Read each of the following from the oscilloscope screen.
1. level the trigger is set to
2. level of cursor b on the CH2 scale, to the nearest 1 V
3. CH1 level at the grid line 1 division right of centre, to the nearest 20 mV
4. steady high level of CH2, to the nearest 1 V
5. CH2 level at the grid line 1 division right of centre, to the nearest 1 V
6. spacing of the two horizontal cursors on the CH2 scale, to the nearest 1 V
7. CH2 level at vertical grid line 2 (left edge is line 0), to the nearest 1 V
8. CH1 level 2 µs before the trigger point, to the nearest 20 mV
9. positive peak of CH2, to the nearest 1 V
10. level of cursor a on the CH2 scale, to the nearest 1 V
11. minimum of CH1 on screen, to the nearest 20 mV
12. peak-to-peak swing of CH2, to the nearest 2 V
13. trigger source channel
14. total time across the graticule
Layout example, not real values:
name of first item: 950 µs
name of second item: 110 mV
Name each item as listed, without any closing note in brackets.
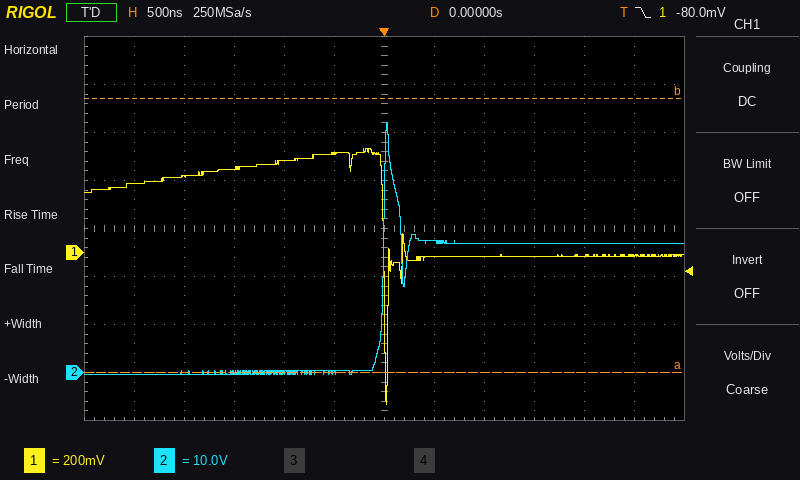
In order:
level the trigger is set to: -80.0 mV
level of cursor b on the CH2 scale, to the nearest 1 V: 57 V
CH1 level at the grid line 1 division right of centre, to the nearest 20 mV: -20 mV
steady high level of CH2, to the nearest 1 V: 27 V
CH2 level at the grid line 1 division right of centre, to the nearest 1 V: 27 V
spacing of the two horizontal cursors on the CH2 scale, to the nearest 1 V: 57 V
CH2 level at vertical grid line 2 (left edge is line 0), to the nearest 1 V: 0 V
CH1 level 2 µs before the trigger point, to the nearest 20 mV: 320 mV
positive peak of CH2, to the nearest 1 V: 52 V
level of cursor a on the CH2 scale, to the nearest 1 V: 0 V
minimum of CH1 on screen, to the nearest 20 mV: -640 mV
peak-to-peak swing of CH2, to the nearest 2 V: 52 V
trigger source channel: CH1
total time across the graticule: 6 µs
